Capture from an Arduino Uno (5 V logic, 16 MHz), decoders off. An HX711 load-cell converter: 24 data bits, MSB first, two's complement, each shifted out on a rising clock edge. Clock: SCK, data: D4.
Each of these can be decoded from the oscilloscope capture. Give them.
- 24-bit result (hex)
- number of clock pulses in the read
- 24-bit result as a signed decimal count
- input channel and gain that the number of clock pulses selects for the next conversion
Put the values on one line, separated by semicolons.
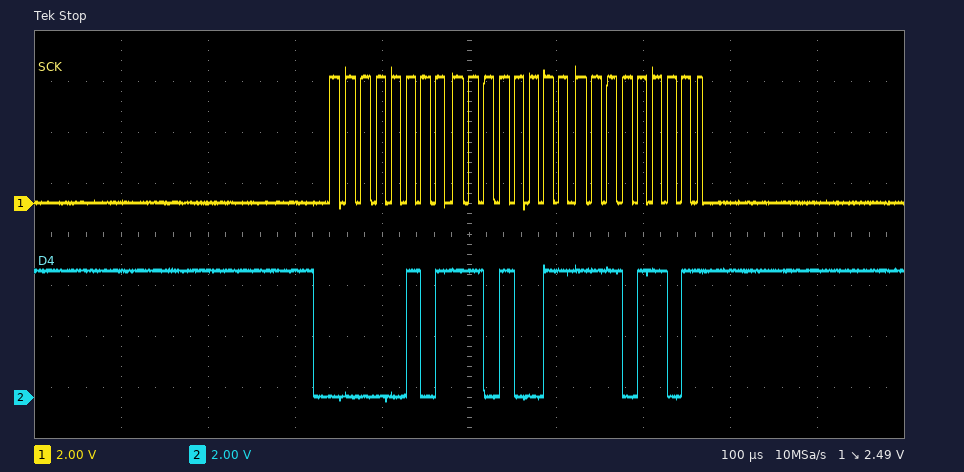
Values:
0x05D3ED; 25; 381933; channel A, gain 128
